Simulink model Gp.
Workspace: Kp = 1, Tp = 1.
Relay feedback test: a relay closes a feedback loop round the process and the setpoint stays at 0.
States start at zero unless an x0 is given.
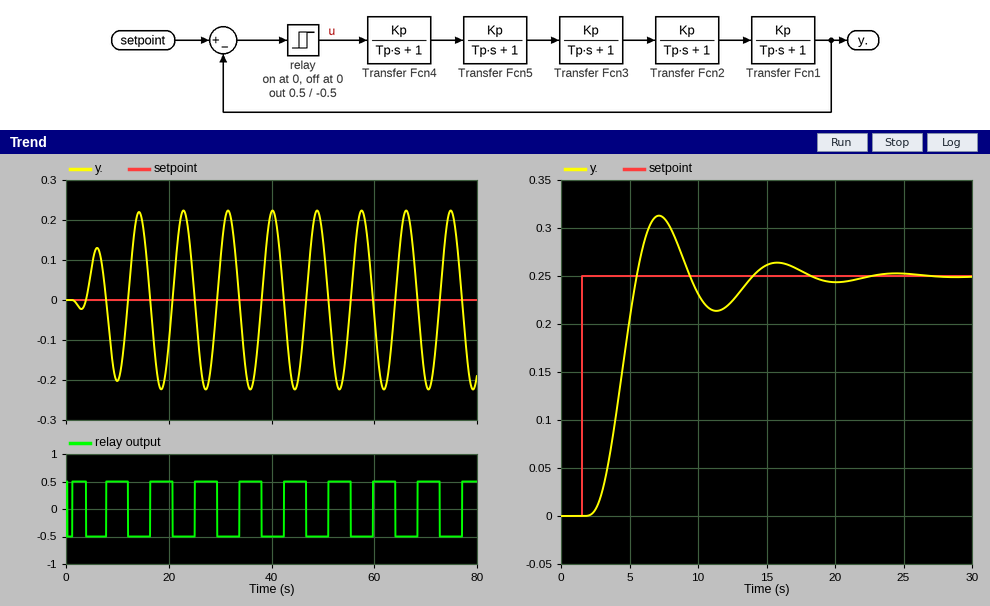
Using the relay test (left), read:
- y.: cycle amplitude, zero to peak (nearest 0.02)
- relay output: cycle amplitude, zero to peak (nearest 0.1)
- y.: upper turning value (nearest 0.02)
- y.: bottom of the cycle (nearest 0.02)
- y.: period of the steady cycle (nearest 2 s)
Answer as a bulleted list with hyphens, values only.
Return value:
- 0.22
- 0.5
- 0.22
- -0.22
- 8 s
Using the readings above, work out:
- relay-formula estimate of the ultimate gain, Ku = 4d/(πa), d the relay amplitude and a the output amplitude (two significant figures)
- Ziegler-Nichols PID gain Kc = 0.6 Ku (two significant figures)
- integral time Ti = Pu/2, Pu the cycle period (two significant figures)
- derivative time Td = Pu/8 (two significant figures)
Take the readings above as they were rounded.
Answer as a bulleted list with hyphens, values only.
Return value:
- 2.9
- 1.7
- 4.0 s
- 1.0 s
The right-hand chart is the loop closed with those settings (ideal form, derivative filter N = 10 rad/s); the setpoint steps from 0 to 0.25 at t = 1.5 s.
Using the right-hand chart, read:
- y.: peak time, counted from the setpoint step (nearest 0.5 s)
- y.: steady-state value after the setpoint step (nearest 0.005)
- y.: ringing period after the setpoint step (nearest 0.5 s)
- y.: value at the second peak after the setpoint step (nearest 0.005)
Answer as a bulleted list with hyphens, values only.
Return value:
- 5.5 s
- 0.250
- 8.5 s
- 0.265
